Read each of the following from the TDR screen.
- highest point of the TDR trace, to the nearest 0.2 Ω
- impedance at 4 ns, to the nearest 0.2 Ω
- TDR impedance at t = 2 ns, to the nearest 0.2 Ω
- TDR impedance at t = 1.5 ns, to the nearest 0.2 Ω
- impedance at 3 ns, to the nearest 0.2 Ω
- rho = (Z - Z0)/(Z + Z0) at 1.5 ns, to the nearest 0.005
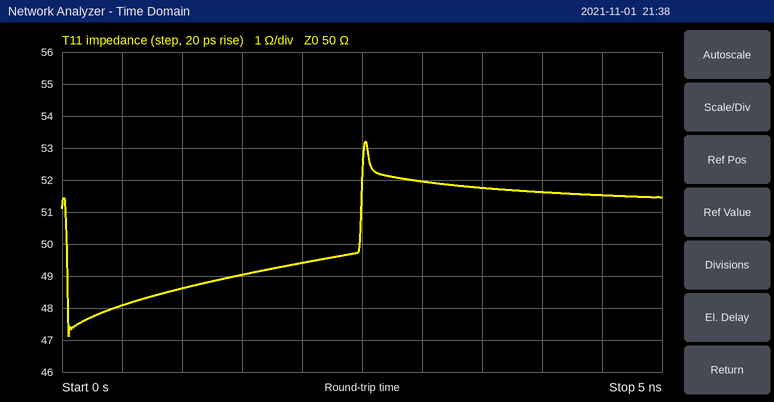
53.2 Ω
51.6 Ω
49.4 Ω
49.0 Ω
52.0 Ω
-0.010
